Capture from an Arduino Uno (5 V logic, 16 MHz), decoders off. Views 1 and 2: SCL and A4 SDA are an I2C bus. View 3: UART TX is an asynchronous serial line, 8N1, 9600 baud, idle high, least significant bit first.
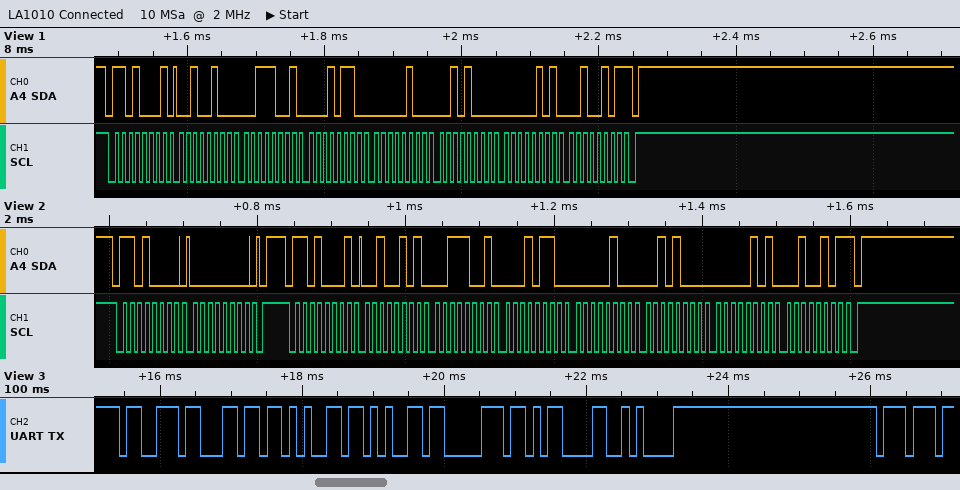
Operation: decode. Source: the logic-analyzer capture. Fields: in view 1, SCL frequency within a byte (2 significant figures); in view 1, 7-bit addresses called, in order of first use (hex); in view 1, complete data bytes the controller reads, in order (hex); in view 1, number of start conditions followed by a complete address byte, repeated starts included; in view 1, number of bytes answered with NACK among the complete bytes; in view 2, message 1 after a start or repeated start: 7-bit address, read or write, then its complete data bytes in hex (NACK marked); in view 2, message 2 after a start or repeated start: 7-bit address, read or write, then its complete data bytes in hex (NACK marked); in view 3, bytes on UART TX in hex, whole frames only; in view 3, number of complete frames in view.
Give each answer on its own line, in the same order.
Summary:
100 kHz
0x68
24 39 16 04 28 05 25
1
1
0x68 write: 00
0x68 read: 25 39 16 04 28 05 25 NACK
73 6C 65 65 70 0D 0A 77
8
